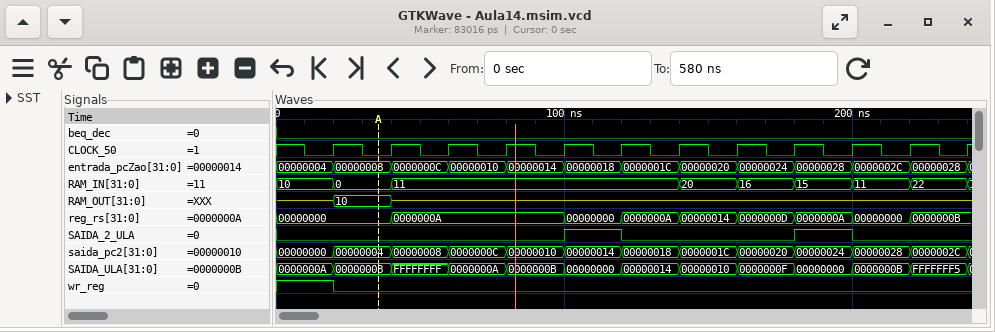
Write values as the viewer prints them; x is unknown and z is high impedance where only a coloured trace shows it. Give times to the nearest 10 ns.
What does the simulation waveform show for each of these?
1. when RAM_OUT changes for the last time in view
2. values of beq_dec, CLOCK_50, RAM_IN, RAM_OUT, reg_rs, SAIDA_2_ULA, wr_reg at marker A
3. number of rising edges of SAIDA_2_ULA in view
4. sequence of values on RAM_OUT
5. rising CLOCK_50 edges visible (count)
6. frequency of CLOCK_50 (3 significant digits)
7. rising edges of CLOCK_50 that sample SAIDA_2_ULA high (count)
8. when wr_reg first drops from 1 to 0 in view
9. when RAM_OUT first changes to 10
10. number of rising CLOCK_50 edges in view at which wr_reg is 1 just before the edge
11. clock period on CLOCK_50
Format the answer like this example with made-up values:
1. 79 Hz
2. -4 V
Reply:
1. 40 ns
2. beq_dec=0, CLOCK_50=0, RAM_IN=0, RAM_OUT=10, reg_rs=00000000, SAIDA_2_ULA=0, wr_reg=0
3. 2
4. z, 10, z
5. 12
6. 50.0 MHz
7. 2
8. 20 ns
9. 20 ns
10. 1
11. 20 ns
